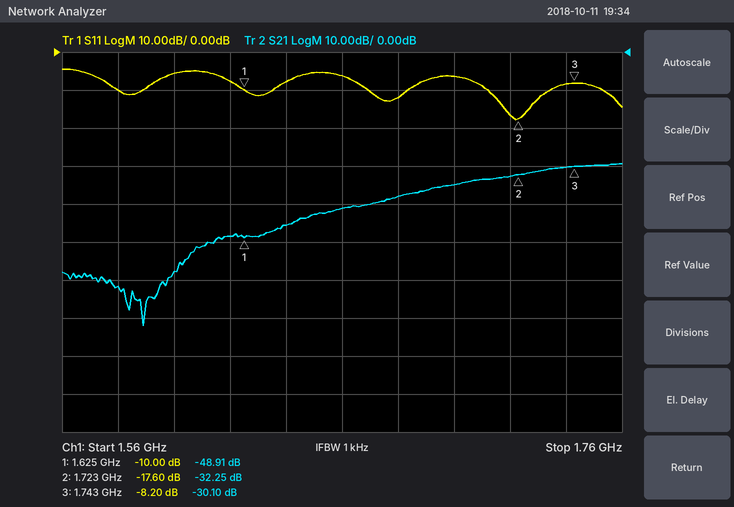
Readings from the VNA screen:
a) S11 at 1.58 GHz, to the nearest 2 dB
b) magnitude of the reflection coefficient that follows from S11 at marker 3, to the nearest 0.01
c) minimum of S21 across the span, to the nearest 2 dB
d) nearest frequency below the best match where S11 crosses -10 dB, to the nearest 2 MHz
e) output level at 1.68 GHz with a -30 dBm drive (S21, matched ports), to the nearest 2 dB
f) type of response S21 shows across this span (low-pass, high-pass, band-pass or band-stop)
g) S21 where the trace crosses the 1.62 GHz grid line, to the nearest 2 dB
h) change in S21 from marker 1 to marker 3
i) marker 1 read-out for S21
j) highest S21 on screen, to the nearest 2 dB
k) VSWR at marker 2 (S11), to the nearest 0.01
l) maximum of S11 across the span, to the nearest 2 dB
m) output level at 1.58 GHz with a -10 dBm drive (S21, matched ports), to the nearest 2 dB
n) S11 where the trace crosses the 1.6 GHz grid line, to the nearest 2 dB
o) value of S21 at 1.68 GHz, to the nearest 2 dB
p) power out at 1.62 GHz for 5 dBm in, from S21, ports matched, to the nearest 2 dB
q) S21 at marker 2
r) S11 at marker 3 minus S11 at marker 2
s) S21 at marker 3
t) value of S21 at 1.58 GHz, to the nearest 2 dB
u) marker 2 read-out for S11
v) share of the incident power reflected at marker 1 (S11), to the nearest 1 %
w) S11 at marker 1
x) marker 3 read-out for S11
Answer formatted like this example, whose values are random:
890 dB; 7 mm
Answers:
-10 dB; 0.39; -72 dB; 1.712 GHz; -68 dBm; high-pass; -48 dB; 18.81 dB; -48.91 dB; -30 dB; 1.30; -4 dB; -72 dBm; -6 dB; -38 dB; -44 dBm; -32.25 dB; 9.40 dB; -30.10 dB; -62 dB; -17.60 dB; 10 %; -10.00 dB; -8.20 dB
